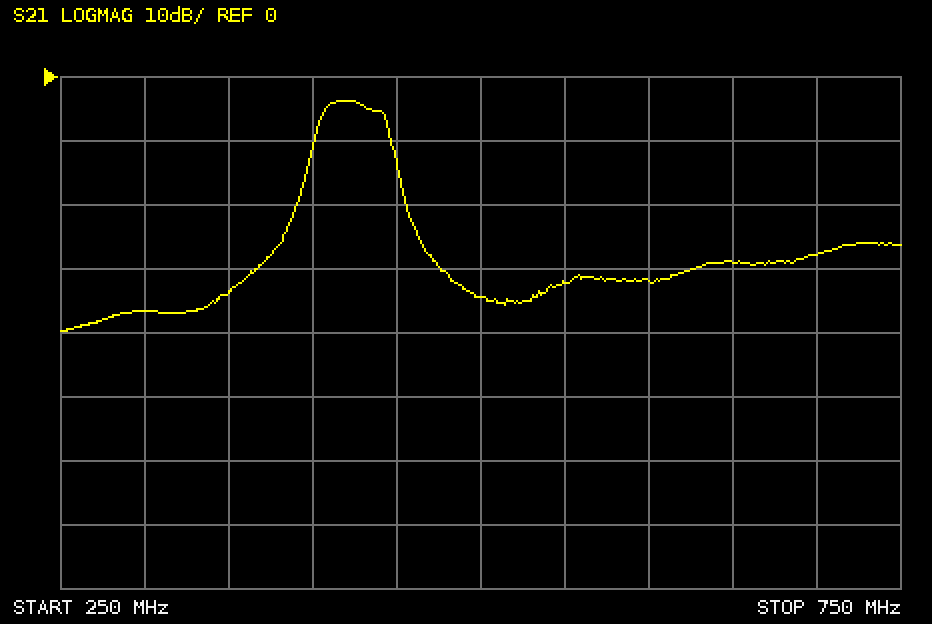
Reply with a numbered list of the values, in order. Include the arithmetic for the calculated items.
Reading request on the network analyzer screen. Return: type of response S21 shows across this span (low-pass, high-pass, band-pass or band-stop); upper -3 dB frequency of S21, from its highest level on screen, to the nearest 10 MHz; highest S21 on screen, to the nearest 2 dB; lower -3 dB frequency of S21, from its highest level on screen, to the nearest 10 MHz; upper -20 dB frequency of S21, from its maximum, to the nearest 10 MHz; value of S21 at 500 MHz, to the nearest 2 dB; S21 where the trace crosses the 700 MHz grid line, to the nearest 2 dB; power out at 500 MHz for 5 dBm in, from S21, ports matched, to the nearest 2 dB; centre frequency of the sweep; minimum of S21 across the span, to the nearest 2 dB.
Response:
1. band-pass
2. 440 MHz
3. -4 dB
4. 400 MHz
5. 460 MHz
6. -34 dB
7. -28 dB
8. 5 dBm + (-34 dB) = -30 dBm
9. 500 MHz
10. -40 dB
